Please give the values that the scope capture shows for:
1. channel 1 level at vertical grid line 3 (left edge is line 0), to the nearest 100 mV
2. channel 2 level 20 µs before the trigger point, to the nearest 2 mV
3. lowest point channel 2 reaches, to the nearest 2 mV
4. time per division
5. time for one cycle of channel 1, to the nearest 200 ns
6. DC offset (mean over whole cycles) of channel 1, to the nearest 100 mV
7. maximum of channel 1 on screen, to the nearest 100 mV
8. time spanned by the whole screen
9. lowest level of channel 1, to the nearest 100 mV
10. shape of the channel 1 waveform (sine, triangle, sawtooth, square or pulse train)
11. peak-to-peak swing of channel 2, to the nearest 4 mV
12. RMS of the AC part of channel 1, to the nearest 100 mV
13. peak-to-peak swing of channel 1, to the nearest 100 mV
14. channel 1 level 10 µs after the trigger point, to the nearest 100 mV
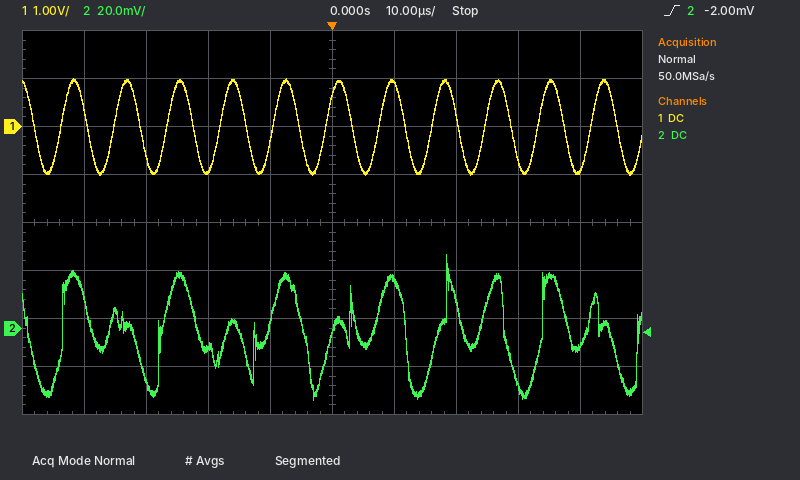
-900 mV
-8 mV
-30 mV
10 µs
8.6 µs
0.0 V
1.0 V
100 µs
-1.0 V
sine
60 mV
700 mV
2.0 V
900 mV
